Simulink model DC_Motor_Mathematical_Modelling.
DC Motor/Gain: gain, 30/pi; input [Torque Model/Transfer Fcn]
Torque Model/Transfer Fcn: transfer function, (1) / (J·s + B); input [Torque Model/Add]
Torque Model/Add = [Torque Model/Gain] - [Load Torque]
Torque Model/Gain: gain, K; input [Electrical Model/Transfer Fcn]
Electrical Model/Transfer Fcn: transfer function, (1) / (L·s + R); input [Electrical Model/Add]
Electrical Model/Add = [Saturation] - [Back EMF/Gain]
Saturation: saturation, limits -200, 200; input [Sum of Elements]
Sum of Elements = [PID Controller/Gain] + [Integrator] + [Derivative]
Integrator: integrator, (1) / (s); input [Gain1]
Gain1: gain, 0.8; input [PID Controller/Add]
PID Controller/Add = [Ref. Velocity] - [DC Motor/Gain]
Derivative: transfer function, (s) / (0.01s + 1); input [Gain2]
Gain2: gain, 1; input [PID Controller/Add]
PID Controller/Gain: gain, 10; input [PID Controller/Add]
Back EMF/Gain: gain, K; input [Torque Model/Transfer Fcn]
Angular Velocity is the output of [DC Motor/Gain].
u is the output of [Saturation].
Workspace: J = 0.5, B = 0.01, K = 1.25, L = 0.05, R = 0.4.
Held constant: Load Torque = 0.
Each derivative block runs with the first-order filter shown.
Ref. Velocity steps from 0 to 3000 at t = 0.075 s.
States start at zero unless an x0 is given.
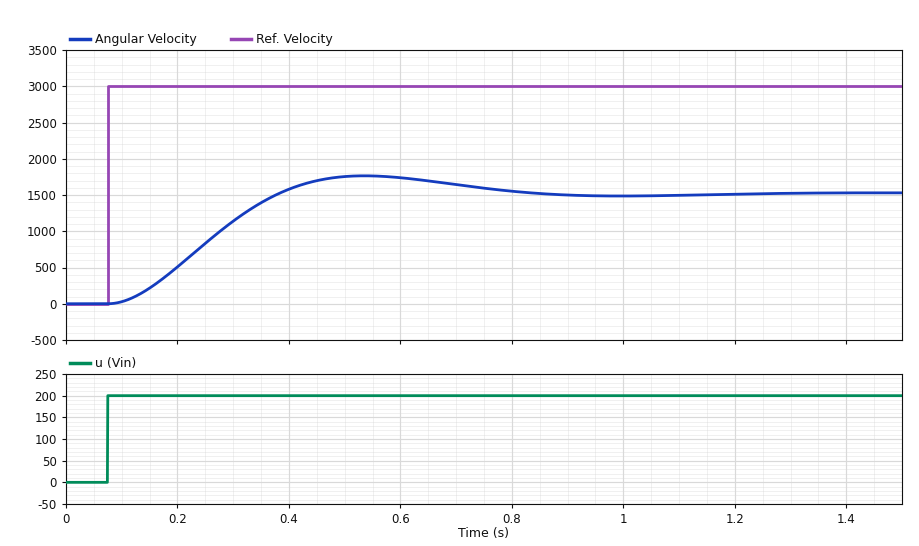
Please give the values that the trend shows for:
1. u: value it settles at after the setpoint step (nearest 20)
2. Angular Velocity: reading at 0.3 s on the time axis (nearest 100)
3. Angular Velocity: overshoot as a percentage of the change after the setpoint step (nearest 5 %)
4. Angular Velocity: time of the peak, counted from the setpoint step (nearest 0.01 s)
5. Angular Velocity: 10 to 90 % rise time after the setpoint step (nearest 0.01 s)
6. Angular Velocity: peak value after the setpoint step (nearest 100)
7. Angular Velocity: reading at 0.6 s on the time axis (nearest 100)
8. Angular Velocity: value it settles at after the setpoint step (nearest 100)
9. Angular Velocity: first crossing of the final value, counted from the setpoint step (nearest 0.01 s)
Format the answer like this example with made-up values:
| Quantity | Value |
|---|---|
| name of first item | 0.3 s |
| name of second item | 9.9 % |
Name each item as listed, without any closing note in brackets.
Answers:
| Quantity | Value |
|---|---|
| u: value it settles at after the setpoint step | 200 |
| Angular Velocity: reading at 0.3 s on the time axis | 1100 |
| Angular Velocity: overshoot as a percentage of the change after the setpoint step | 15 % |
| Angular Velocity: time of the peak, counted from the setpoint step | 0.46 s |
| Angular Velocity: 10 to 90 % rise time after the setpoint step | 0.21 s |
| Angular Velocity: peak value after the setpoint step | 1800 |
| Angular Velocity: reading at 0.6 s on the time axis | 1700 |
| Angular Velocity: value it settles at after the setpoint step | 1500 |
| Angular Velocity: first crossing of the final value, counted from the setpoint step | 0.31 s |
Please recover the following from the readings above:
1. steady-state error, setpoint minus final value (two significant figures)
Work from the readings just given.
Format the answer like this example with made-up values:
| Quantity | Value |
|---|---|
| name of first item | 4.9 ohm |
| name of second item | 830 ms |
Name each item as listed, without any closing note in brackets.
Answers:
| Quantity | Value |
|---|---|
| steady-state error, setpoint minus final value | 1500 |
